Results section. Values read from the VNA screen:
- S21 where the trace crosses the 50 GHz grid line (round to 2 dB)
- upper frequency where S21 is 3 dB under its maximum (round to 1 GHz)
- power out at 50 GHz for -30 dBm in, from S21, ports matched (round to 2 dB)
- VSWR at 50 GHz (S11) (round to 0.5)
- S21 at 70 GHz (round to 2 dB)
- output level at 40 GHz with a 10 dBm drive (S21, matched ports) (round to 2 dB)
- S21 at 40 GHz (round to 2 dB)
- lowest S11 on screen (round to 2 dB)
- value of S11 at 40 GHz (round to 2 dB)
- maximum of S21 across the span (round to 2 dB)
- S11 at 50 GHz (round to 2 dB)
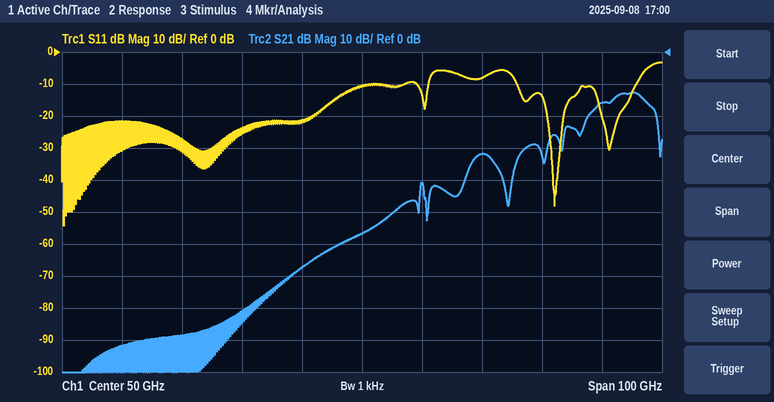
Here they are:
-56 dB
97 GHz
-86 dBm
2.0
-32 dB
-58 dBm
-68 dB
-54 dB
-22 dB
-12 dB
-10 dB
